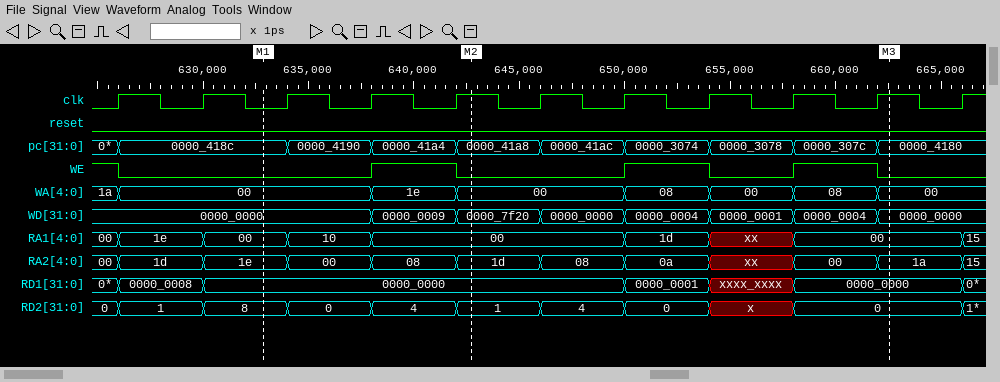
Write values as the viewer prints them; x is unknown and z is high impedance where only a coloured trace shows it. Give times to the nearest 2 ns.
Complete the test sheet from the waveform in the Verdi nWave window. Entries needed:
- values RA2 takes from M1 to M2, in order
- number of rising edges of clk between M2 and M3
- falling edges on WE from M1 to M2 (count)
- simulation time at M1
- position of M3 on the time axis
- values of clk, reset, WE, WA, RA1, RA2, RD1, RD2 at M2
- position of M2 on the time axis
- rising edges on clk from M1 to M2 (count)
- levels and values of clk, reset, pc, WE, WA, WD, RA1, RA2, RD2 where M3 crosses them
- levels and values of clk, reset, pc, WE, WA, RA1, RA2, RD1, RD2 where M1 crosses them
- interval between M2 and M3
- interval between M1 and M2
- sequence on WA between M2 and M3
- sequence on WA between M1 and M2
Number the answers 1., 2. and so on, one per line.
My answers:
1. 1e, 00, 08, 1d
2. 5
3. 1
4. 632 ns
5. 662 ns
6. clk=1, reset=0, WE=0, WA=00, RA1=00, RA2=1d, RD1=0000_0000, RD2=1
7. 642 ns
8. 3
9. clk=1, reset=0, pc=0000_4180, WE=0, WA=00, WD=0000_0000, RA1=00, RA2=1a, RD2=0
10. clk=0, reset=0, pc=0000_418c, WE=0, WA=00, RA1=00, RA2=1e, RD1=0000_0000, RD2=8
11. 20 ns
12. 10 ns
13. 00, 08, 00, 08, 00
14. 00, 1e, 00
